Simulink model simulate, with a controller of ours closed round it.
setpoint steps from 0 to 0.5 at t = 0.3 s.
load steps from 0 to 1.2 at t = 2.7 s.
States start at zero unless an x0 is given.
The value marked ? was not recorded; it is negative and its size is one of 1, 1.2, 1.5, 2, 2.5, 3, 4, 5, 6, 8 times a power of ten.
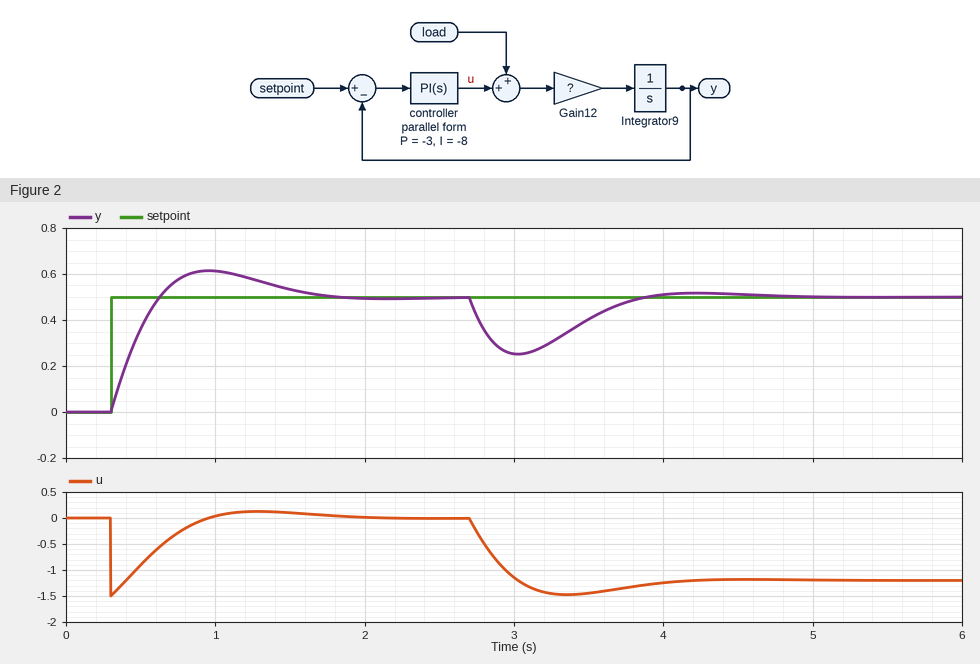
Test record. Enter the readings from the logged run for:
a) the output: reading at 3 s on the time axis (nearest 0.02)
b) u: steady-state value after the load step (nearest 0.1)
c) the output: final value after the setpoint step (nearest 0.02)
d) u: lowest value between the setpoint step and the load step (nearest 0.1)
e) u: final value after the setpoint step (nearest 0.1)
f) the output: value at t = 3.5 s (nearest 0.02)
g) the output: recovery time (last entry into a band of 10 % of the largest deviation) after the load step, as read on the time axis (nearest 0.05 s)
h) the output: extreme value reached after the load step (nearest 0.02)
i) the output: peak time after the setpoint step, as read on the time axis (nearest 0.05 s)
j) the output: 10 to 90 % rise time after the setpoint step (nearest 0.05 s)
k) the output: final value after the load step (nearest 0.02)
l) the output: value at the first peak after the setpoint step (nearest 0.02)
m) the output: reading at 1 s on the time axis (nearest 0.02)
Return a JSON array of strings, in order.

["0.26", "-1.2", "0.50", "-1.5", "0.0", "0.40", "3.75 s", "0.26", "0.95 s", "0.25 s", "0.50", "0.62", "0.62"]
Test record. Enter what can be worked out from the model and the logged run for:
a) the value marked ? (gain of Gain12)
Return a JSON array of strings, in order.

["-1.5"]
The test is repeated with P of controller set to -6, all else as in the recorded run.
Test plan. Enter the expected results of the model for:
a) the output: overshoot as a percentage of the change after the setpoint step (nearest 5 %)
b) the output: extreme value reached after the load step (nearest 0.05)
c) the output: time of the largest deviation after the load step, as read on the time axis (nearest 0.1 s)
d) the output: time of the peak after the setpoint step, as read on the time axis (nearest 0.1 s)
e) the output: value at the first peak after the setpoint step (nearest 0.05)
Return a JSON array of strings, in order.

["10 %", "0.35", "3.0 s", "0.8 s", "0.55"]
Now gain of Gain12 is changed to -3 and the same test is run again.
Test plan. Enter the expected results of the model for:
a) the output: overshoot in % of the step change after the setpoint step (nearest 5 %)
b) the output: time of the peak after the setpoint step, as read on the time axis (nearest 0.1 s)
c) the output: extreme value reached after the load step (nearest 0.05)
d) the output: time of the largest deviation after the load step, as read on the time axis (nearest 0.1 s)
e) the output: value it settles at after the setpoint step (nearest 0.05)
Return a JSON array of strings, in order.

["15 %", "0.7 s", "0.20", "2.9 s", "0.50"]
